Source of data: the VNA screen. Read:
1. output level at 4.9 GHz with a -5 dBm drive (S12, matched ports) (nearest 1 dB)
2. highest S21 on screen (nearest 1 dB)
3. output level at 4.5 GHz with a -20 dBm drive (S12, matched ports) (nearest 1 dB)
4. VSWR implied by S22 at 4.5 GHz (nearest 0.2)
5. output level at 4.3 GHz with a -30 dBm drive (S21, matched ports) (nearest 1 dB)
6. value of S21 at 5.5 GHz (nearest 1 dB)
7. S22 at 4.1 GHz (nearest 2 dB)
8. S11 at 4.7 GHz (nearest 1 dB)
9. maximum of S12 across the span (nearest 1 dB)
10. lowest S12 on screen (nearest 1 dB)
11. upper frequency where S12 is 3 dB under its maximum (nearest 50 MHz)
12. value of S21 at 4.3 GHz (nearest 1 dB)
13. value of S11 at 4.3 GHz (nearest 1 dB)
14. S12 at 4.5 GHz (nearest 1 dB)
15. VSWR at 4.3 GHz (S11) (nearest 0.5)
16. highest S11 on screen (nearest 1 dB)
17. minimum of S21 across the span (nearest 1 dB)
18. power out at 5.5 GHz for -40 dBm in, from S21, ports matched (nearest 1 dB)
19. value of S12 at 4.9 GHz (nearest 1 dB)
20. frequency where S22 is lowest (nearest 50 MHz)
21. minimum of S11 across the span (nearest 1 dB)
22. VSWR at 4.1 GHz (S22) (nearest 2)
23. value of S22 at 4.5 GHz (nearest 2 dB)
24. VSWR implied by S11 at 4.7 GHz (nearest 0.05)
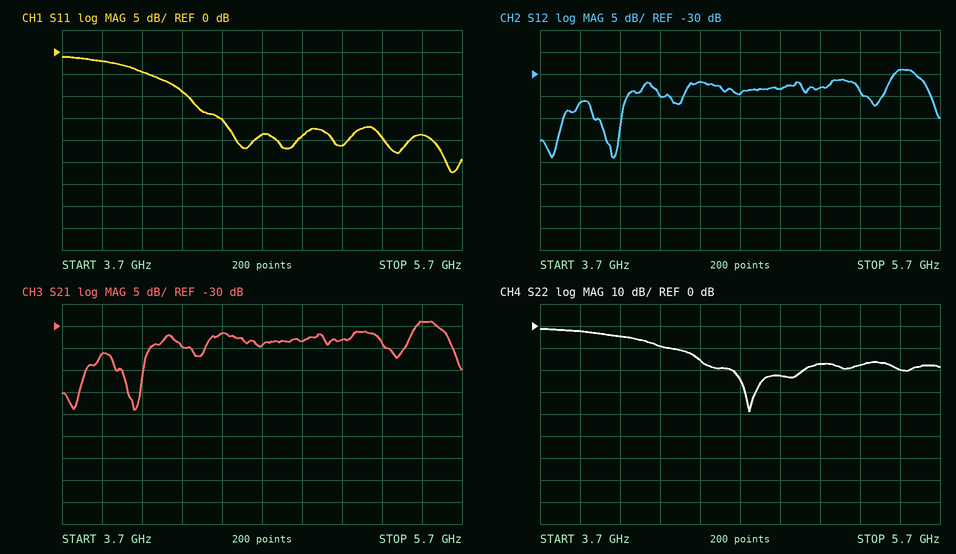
-38 dBm
-29 dB
-52 dBm
1.4
-65 dBm
-29 dB
-4 dB
-19 dB
-29 dB
-49 dB
5.60 GHz
-35 dB
-9 dB
-32 dB
2.0
-1 dB
-49 dB
-69 dBm
-33 dB
4.75 GHz
-27 dB
4
-16 dB
1.25
